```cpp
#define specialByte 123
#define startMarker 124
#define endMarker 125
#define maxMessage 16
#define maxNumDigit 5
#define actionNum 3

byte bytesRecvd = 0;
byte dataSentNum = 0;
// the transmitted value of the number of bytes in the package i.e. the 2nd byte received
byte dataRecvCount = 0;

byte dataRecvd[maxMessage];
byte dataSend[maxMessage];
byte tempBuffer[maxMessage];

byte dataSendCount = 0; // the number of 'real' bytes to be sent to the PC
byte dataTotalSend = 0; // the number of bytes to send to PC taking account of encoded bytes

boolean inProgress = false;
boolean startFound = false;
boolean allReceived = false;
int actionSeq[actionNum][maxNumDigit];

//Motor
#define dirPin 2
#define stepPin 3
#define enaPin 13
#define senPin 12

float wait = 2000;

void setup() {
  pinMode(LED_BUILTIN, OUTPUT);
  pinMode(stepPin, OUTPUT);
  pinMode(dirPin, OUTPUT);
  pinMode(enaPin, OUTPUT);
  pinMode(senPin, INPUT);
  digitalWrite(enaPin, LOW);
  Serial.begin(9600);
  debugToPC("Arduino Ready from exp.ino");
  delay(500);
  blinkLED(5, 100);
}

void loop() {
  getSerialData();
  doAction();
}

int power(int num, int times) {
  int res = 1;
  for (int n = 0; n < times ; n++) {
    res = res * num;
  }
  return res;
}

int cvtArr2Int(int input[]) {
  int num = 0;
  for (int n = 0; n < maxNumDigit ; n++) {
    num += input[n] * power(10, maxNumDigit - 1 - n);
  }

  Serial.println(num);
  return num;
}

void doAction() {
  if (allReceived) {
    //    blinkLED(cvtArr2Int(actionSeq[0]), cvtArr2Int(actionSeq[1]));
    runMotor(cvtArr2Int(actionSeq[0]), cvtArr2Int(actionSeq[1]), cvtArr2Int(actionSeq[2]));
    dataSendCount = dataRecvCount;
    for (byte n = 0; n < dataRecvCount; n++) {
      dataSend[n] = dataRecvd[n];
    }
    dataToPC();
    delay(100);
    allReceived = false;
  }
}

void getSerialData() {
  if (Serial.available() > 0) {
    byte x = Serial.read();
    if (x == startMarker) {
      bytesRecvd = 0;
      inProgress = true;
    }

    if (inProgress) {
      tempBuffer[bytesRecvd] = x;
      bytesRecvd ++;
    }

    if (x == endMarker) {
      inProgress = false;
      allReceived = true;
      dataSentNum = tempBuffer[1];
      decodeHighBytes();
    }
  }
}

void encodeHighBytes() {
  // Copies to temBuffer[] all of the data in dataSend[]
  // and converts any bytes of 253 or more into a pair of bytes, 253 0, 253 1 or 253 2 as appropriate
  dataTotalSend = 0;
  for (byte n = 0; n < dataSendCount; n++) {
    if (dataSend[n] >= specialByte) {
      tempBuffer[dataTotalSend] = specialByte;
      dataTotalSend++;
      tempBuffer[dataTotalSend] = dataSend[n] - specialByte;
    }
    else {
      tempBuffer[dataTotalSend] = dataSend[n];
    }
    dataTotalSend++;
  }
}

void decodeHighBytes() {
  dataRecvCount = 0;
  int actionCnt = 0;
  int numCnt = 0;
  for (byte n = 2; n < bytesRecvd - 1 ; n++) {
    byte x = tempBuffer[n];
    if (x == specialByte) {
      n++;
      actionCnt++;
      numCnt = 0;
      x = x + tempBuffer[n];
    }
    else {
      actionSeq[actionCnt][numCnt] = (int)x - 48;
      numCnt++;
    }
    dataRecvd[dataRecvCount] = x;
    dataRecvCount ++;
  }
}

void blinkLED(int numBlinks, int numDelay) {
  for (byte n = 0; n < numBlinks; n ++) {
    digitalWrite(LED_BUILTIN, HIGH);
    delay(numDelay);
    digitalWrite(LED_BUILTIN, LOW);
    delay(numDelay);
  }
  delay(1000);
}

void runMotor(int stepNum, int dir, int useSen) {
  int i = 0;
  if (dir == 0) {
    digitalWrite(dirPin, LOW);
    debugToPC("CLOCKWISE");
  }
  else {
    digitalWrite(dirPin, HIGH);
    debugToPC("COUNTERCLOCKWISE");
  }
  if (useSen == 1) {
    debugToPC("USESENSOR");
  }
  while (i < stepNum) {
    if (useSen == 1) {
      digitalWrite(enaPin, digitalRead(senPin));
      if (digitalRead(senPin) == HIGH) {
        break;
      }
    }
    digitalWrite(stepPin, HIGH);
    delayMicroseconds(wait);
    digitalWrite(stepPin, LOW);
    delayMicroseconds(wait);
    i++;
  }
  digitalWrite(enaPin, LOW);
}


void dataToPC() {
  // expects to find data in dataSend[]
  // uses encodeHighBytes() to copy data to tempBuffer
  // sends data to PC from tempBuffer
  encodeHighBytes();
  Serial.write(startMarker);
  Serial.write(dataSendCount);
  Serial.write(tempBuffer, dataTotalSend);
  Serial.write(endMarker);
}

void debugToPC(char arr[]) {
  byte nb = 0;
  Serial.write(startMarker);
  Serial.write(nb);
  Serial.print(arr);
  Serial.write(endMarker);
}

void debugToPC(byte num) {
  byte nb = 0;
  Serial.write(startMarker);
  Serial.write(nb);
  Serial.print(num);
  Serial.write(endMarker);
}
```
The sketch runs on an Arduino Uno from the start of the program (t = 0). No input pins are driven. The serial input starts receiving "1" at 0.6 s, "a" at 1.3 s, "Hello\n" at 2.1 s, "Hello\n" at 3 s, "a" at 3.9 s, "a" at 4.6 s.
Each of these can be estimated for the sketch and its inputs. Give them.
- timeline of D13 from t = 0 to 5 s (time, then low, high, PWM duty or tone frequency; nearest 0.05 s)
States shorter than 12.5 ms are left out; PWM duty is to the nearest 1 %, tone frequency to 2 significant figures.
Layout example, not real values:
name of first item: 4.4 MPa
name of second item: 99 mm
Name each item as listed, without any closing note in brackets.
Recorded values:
timeline of D13 from t = 0 to 5 s: 0 s low; 0.5 s high; 0.6 s low; 0.7 s high; 0.8 s low; 0.9 s high; 1 s low; 1.1 s high; 1.2 s low; 1.3 s high; 1.4 s low
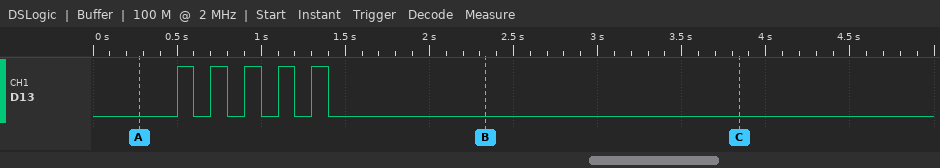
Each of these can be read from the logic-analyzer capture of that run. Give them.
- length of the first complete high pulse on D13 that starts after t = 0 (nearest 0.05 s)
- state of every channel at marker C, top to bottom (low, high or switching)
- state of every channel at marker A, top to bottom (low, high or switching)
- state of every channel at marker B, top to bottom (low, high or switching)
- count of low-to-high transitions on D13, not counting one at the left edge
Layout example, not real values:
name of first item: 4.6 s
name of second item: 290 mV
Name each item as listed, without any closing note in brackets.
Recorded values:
length of the first complete high pulse on D13 that starts after t = 0: 0.10 s
state of every channel at marker C, top to bottom: D13 low
state of every channel at marker A, top to bottom: D13 low
state of every channel at marker B, top to bottom: D13 low
count of low-to-high transitions on D13, not counting one at the left edge: 5
